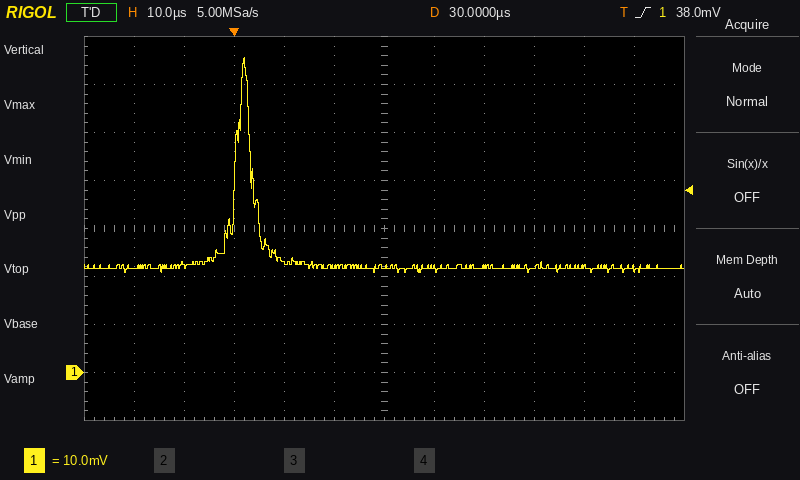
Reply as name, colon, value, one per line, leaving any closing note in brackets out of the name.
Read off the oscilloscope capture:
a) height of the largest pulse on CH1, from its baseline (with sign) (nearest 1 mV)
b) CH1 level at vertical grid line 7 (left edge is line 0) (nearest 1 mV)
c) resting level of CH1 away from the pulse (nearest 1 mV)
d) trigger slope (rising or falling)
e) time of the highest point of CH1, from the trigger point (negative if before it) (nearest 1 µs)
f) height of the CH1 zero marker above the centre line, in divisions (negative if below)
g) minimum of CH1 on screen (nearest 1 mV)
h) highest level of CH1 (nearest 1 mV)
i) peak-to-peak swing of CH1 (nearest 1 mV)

height of the largest pulse on CH1, from its baseline (with sign): +44 mV
CH1 level at vertical grid line 7 (left edge is line 0): 22 mV
resting level of CH1 away from the pulse: 22 mV
trigger slope: rising
time of the highest point of CH1, from the trigger point (negative if before it): +2 µs
height of the CH1 zero marker above the centre line, in divisions: -3.0 div
minimum of CH1 on screen: 21 mV
highest level of CH1: 66 mV
peak-to-peak swing of CH1: 45 mV
